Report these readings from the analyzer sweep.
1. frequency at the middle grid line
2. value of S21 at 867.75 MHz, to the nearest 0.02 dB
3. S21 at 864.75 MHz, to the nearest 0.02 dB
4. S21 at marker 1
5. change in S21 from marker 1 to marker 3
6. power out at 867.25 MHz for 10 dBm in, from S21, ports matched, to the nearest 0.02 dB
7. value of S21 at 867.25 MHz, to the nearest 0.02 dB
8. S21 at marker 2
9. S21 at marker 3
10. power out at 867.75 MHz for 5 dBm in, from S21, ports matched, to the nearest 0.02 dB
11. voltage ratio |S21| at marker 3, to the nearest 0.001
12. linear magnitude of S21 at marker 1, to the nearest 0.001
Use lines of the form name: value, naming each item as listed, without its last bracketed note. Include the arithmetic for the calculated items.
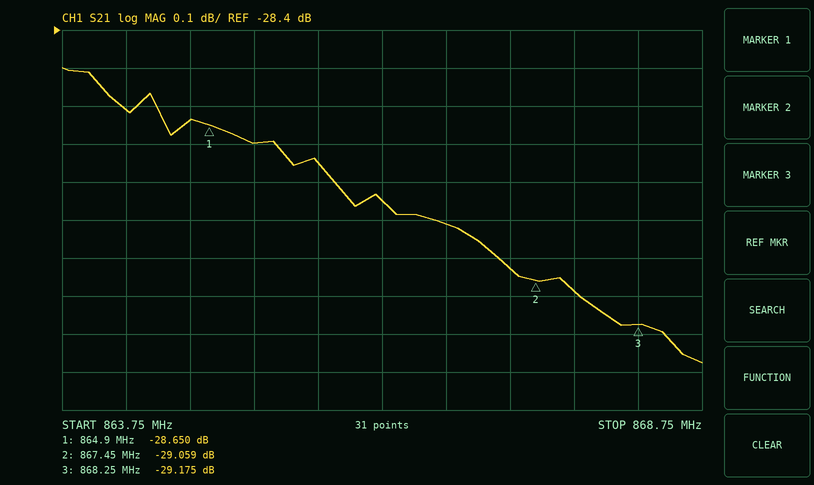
frequency at the middle grid line: 866.25 MHz
value of S21 at 867.75 MHz, to the nearest 0.02 dB: -29.08 dB
S21 at 864.75 MHz, to the nearest 0.02 dB: -28.64 dB
S21 at marker 1: -28.650 dB
change in S21 from marker 1 to marker 3: -29.175 − (-28.65) = -0.525 dB
power out at 867.25 MHz for 10 dBm in, from S21, ports matched, to the nearest 0.02 dB: 10 dBm + (-29.02 dB) = -19.02 dBm
value of S21 at 867.25 MHz, to the nearest 0.02 dB: -29.02 dB
S21 at marker 2: -29.059 dB
S21 at marker 3: -29.175 dB
power out at 867.75 MHz for 5 dBm in, from S21, ports matched, to the nearest 0.02 dB: 5 dBm + (-29.08 dB) = -24.08 dBm
voltage ratio |S21| at marker 3, to the nearest 0.001: 10^(-29.175/20) ≈ 0.035
linear magnitude of S21 at marker 1, to the nearest 0.001: 10^(-28.65/20) ≈ 0.037
